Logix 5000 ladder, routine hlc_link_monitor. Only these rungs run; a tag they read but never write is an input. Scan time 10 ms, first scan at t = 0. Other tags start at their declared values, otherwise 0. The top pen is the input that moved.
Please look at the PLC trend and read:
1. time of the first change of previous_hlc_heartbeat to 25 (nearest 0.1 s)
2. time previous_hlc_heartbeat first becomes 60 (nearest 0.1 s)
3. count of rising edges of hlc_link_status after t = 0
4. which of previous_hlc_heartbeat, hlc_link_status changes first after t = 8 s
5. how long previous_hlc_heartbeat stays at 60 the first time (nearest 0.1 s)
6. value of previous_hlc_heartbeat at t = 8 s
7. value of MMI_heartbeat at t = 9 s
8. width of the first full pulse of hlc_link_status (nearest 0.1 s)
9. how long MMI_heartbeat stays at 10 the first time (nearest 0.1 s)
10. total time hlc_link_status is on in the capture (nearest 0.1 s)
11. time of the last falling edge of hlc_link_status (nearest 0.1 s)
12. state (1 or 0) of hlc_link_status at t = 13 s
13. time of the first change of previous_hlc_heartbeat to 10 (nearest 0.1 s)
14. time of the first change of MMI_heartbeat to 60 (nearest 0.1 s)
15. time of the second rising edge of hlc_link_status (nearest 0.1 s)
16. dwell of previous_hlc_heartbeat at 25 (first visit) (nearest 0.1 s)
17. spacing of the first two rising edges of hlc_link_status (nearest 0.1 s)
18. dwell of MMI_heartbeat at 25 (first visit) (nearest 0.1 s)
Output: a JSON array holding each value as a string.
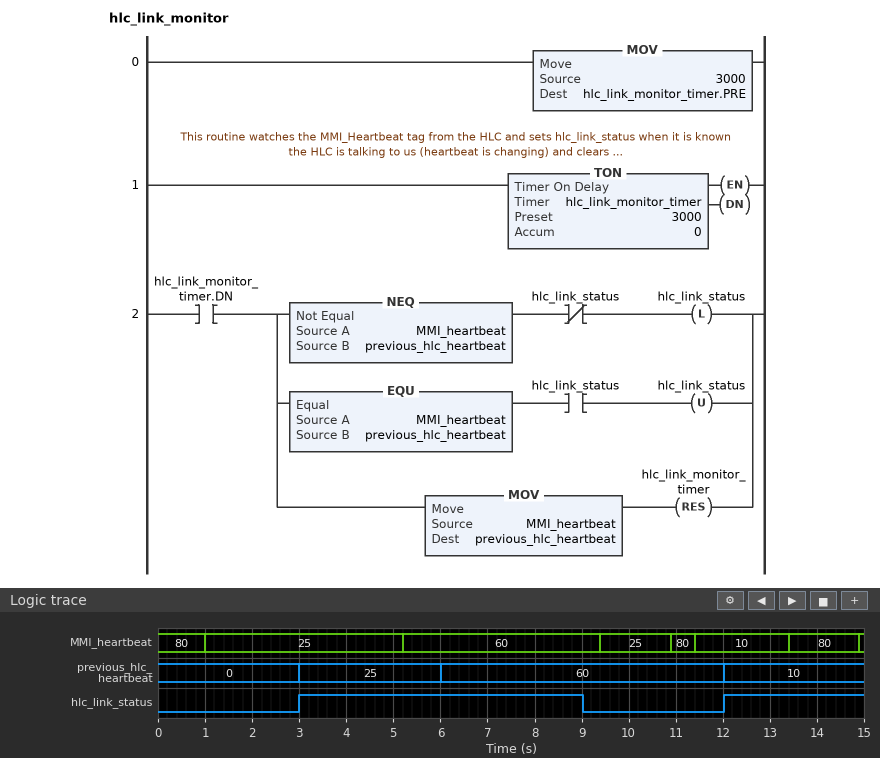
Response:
["3.0 s", "6.0 s", "2", "hlc_link_status", "6.0 s", "60", "60", "6.0 s", "2.0 s", "9.0 s", "9.0 s", "1", "12.0 s", "5.2 s", "12.0 s", "3.0 s", "9.0 s", "4.2 s"]
